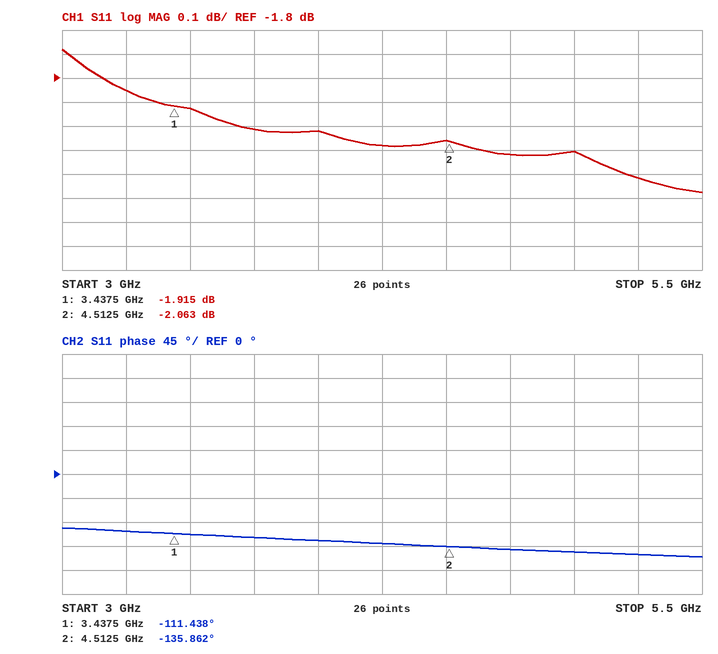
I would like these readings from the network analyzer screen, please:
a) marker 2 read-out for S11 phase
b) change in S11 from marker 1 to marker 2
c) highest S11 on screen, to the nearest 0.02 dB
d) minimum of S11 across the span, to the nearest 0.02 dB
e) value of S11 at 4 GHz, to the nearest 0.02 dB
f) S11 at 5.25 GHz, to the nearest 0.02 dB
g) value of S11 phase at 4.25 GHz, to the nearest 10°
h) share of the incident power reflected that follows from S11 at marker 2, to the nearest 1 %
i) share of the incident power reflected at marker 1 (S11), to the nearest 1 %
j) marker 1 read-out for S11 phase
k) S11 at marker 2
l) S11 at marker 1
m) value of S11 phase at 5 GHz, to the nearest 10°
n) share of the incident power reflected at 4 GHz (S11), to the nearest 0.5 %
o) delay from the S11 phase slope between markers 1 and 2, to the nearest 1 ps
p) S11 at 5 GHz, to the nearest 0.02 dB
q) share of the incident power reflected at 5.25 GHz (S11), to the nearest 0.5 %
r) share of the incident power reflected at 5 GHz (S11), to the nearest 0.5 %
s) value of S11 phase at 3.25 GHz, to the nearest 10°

-135.862°
-0.148 dB
-1.68 dB
-2.28 dB
-2.02 dB
-2.22 dB
-130°
62 %
64 %
-111.438°
-2.063 dB
-1.915 dB
-150°
63.0 %
63 ps
-2.10 dB
60.0 %
61.5 %
-110°
